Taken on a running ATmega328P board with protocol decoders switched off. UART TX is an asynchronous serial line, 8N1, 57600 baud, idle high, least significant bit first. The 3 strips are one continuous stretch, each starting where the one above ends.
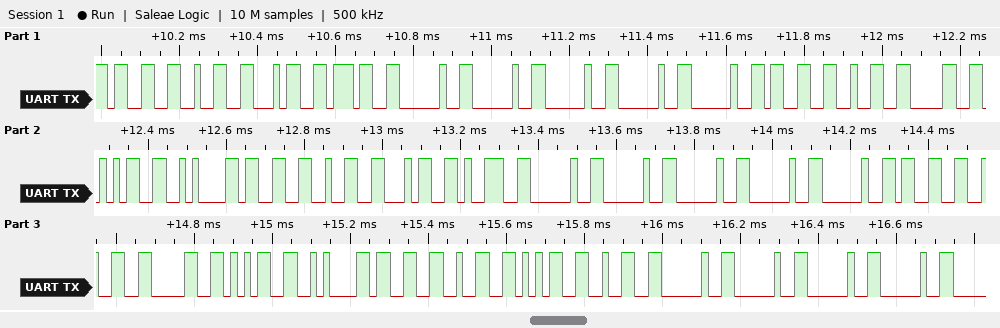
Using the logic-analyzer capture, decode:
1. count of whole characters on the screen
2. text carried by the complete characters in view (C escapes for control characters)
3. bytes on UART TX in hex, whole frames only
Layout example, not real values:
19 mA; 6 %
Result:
36; "3247     3205\n3249     3205\n3252    "; 33 32 34 37 20 20 20 20 20 33 32 30 35 0A 33 32 34 39 20 20 20 20 20 33 32 30 35 0A 33 32 35 32 20 20 20 20
